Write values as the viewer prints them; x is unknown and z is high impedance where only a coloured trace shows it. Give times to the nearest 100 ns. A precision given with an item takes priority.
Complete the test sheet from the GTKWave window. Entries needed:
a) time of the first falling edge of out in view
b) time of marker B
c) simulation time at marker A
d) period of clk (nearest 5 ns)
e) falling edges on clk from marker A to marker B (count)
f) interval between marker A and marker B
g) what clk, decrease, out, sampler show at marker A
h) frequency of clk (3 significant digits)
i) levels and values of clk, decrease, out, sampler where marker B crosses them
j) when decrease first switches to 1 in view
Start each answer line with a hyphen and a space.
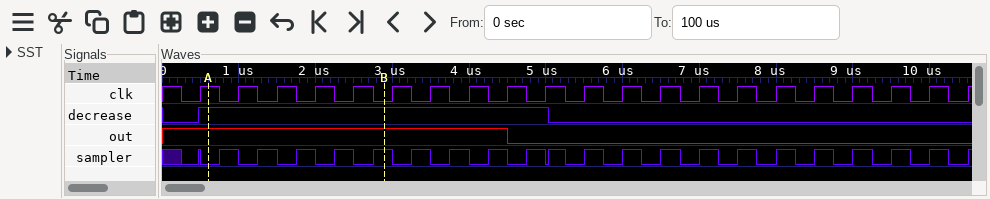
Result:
- 4500 ns
- 2900 ns
- 600 ns
- 500 ns
- 5
- 2300 ns
- clk=1, decrease=1, out=1, sampler=0
- 2.00 MHz
- clk=0, decrease=1, out=1, sampler=1
- 500 ns
